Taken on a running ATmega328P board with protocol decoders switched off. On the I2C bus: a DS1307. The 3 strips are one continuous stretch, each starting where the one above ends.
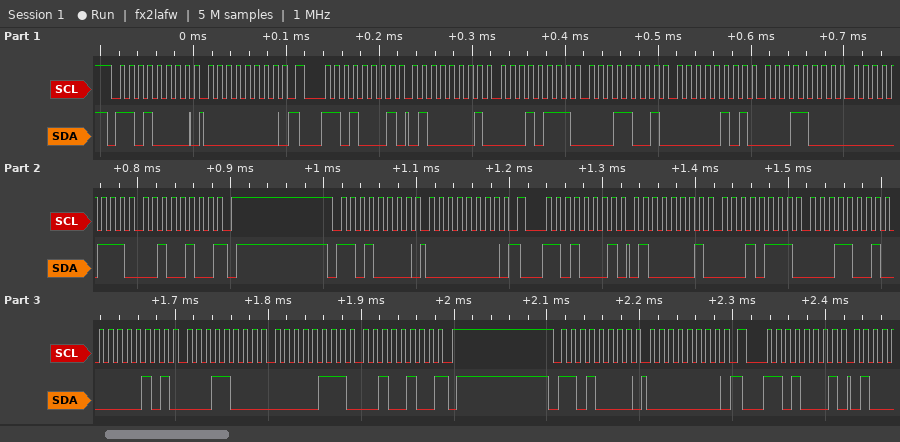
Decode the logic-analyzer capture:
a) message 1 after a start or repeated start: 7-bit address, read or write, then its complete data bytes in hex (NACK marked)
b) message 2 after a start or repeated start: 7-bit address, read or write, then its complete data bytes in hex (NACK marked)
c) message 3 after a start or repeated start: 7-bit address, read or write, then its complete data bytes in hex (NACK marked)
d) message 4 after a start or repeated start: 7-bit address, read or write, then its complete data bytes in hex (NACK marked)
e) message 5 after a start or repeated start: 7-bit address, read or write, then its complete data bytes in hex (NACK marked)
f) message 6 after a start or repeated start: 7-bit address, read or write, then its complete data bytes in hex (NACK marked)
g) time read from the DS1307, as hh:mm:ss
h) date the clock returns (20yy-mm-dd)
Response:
0x68 write: 00
0x68 read: 41 17 19 05 18 07 24 NACK
0x68 write: 00
0x68 read: 41 17 19 05 18 07 24 NACK
0x68 write: 00
0x68 read
19:17:41
2024-07-18
